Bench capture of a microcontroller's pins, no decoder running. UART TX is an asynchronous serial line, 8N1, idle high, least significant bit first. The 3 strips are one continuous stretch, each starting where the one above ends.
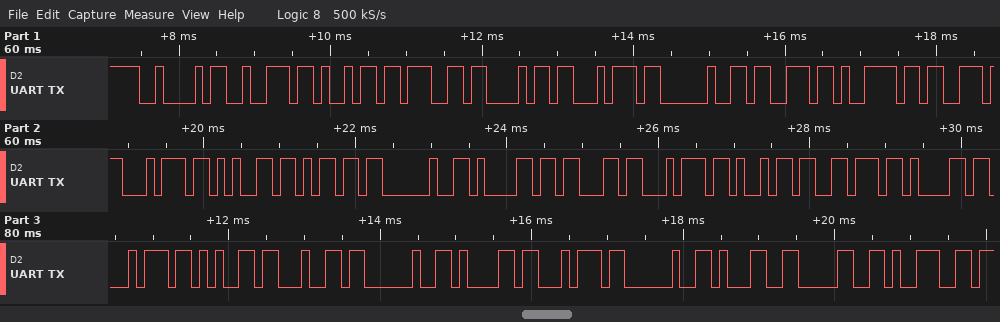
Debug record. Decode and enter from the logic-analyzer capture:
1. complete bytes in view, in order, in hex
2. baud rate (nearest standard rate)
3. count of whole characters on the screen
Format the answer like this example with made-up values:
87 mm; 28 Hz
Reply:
42 72 69 67 68 74 20 73 79 73 74 65 6D 20 61 63 74 69 76 61 74 65 64 20 61 74 20 31 30 39; 9600 baud; 30
